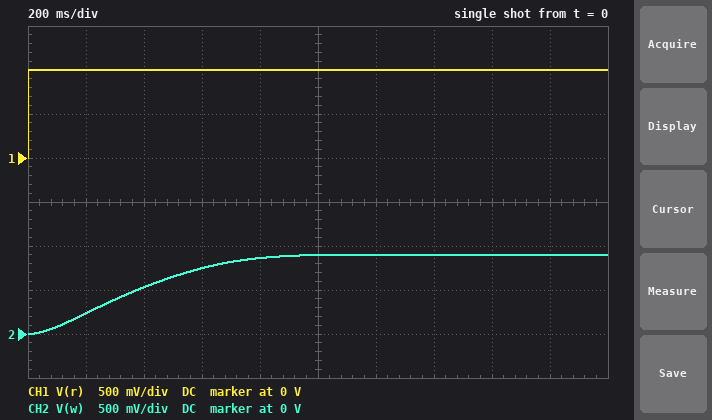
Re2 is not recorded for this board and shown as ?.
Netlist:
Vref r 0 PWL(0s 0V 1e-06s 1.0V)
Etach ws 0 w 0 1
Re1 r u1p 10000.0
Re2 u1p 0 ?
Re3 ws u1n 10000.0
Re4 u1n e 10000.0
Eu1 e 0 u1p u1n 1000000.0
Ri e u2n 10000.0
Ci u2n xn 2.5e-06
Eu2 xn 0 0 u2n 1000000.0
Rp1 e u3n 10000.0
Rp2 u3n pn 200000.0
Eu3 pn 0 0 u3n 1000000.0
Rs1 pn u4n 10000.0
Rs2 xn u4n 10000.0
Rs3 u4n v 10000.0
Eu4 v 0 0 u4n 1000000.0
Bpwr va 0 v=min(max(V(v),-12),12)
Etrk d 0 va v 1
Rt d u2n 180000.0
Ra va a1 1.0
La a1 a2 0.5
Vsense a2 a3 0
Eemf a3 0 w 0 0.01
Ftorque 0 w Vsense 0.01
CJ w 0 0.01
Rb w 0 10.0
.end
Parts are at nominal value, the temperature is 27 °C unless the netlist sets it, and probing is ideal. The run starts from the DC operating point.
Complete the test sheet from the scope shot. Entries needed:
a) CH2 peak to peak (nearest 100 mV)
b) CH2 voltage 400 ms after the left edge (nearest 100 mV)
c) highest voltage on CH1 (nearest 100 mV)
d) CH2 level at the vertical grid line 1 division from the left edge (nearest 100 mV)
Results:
900 mV
500 mV
1.0 V
200 mV
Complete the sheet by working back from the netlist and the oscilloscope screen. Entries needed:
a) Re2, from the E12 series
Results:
8.2 kΩ
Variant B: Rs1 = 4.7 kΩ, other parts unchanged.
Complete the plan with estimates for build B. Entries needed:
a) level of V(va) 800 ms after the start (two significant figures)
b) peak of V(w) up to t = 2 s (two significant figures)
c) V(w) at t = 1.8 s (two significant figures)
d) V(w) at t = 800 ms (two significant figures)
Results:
7.5 V
840 mV
830 mV
760 mV
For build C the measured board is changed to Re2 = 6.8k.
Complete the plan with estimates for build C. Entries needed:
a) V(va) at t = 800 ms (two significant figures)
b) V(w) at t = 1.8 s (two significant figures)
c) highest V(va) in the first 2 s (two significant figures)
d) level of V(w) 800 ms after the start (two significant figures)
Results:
8.3 V
810 mV
12 V
800 mV
